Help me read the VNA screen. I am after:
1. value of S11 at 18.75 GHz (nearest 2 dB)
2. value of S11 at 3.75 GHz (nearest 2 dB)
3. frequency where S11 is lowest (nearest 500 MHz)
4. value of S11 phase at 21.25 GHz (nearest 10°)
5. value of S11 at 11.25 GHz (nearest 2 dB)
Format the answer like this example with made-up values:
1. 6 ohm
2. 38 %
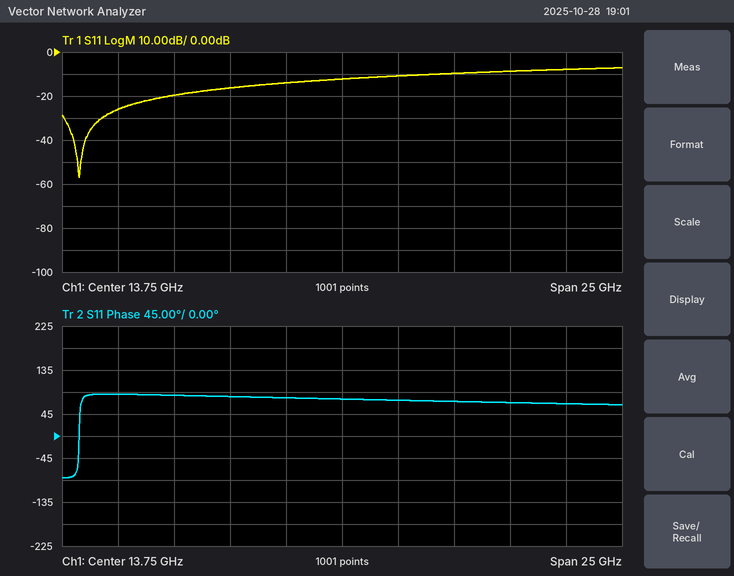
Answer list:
1. -10 dB
2. -26 dB
3. 2.0 GHz
4. 70°
5. -14 dB
